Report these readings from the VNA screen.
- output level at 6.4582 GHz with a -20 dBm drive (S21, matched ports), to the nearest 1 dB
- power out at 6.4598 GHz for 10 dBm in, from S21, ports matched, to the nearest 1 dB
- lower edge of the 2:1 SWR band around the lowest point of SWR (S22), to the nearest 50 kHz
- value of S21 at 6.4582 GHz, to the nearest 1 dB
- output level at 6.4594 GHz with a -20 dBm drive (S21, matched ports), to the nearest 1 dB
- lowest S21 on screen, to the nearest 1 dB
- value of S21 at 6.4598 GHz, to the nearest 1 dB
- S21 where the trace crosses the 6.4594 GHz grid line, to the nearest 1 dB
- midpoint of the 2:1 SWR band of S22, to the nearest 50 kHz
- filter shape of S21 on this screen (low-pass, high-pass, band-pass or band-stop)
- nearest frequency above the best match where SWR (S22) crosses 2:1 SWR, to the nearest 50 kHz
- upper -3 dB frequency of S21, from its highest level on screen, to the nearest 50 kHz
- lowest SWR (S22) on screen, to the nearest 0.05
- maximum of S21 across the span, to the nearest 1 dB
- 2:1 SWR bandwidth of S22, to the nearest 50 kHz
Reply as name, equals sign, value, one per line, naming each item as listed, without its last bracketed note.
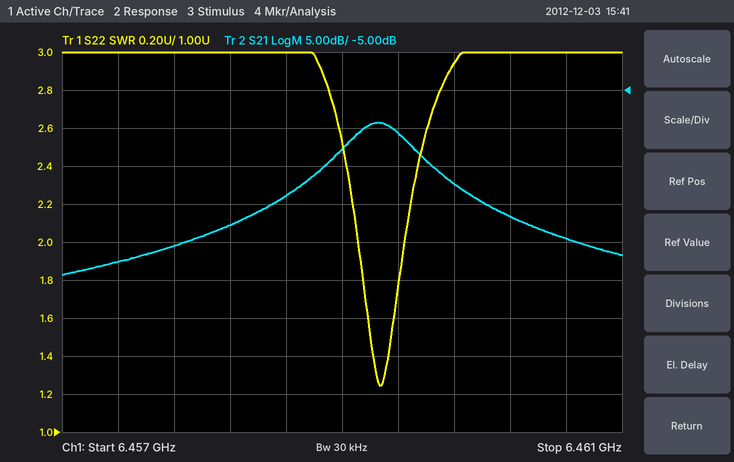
output level at 6.4582 GHz with a -20 dBm drive (S21, matched ports), to the nearest 1 dB = -43 dBm
power out at 6.4598 GHz for 10 dBm in, from S21, ports matched, to the nearest 1 dB = -7 dBm
lower edge of the 2:1 SWR band around the lowest point of SWR (S22), to the nearest 50 kHz = 6.45910 GHz
value of S21 at 6.4582 GHz, to the nearest 1 dB = -23 dB
output level at 6.4594 GHz with a -20 dBm drive (S21, matched ports), to the nearest 1 dB = -31 dBm
lowest S21 on screen, to the nearest 1 dB = -29 dB
value of S21 at 6.4598 GHz, to the nearest 1 dB = -17 dB
S21 where the trace crosses the 6.4594 GHz grid line, to the nearest 1 dB = -11 dB
midpoint of the 2:1 SWR band of S22, to the nearest 50 kHz = 6.45930 GHz
filter shape of S21 on this screen = band-pass
nearest frequency above the best match where SWR (S22) crosses 2:1 SWR, to the nearest 50 kHz = 6.45945 GHz
upper -3 dB frequency of S21, from its highest level on screen, to the nearest 50 kHz = 6.45950 GHz
lowest SWR (S22) on screen, to the nearest 0.05 = 1.25
maximum of S21 across the span, to the nearest 1 dB = -9 dB
2:1 SWR bandwidth of S22, to the nearest 50 kHz = 350 kHz
